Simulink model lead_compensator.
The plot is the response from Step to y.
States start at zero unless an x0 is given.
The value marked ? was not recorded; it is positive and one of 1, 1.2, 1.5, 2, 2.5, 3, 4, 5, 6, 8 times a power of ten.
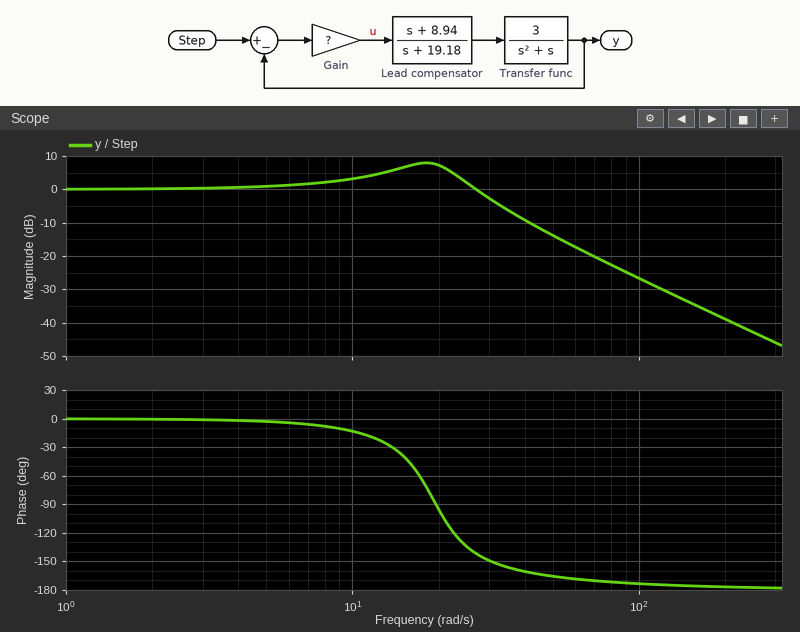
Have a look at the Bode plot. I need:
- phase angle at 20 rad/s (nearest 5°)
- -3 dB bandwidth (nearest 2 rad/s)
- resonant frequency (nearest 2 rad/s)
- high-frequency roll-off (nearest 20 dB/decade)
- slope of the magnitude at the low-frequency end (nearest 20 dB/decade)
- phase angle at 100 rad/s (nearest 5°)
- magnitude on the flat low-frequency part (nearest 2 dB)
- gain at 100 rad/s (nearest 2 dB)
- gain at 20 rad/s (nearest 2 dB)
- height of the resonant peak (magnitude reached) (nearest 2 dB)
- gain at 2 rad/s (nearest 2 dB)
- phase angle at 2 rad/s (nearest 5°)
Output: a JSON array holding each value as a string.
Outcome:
["-95°", "30 rad/s", "18 rad/s", "-40 dB/decade", "0 dB/decade", "-175°", "0 dB", "-26 dB", "8 dB", "8 dB", "0 dB", "0°"]
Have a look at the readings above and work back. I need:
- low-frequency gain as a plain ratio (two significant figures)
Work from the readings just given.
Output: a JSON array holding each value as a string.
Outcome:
["1.0"]
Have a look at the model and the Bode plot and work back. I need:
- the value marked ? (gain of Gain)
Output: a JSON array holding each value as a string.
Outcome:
["150"]
